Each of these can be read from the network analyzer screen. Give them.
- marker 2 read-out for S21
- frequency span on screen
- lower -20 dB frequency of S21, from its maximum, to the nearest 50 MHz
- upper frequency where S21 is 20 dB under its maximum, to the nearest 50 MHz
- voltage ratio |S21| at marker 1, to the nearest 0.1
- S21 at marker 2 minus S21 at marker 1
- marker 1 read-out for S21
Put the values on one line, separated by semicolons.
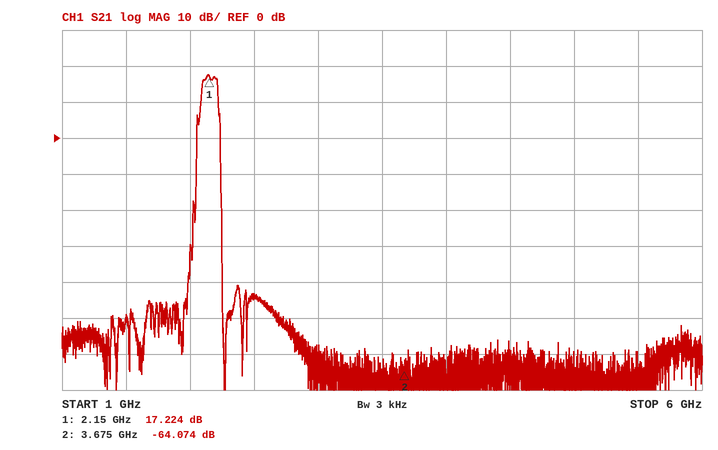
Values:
-64.074 dB; 5 GHz; 2.05 GHz; 2.25 GHz; 7.3; -81.298 dB; 17.224 dB
